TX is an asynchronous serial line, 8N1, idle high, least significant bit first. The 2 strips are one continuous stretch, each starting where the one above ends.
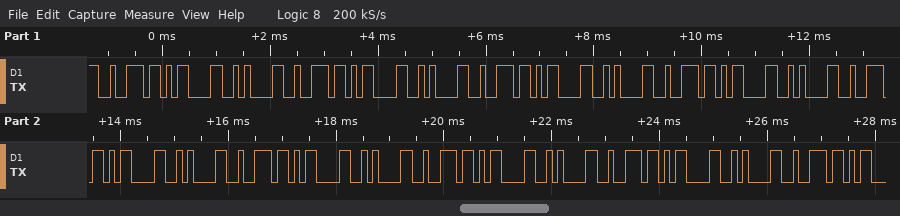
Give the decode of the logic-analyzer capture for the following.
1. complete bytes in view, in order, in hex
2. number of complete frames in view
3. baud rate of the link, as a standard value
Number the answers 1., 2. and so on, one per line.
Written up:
1. 0x72 0x0D 0x0A 0x72 0x0D 0x0A 0x72 0x0D 0x0A 0x72 0x0D 0x0A 0x72 0x0D 0x0A 0x72 0x0D 0x0A 0x72 0x0D 0x0A 0x72 0x0D 0x0A 0x72
2. 25
3. 9600 baud
